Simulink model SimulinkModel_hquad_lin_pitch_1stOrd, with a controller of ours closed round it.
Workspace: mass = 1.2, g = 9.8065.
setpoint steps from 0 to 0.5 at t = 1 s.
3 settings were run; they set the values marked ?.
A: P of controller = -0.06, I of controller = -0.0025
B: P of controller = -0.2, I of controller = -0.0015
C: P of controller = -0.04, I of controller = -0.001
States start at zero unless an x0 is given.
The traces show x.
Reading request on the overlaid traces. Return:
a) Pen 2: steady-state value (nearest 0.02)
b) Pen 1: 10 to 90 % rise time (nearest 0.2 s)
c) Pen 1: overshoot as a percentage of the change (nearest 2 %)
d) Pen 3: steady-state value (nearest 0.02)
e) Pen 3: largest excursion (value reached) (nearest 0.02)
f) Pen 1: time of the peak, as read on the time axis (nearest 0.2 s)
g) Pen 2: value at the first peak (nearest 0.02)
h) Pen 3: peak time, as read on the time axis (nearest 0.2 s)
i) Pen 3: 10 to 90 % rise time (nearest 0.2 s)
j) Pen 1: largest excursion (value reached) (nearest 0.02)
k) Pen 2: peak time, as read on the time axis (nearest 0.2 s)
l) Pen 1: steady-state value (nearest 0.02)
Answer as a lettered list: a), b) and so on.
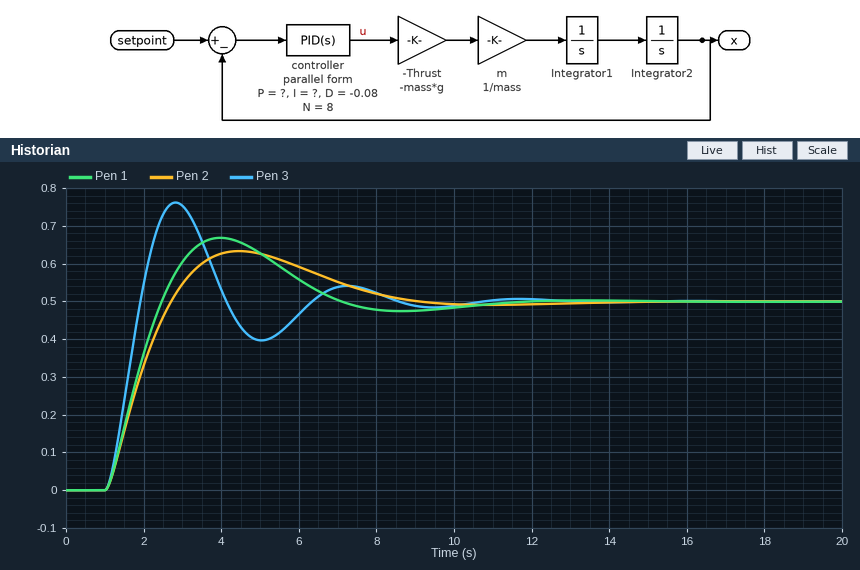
a) 0.50
b) 1.0 s
c) 34 %
d) 0.50
e) 0.76
f) 4.0 s
g) 0.64
h) 2.8 s
i) 0.6 s
j) 0.66
k) 4.4 s
l) 0.50
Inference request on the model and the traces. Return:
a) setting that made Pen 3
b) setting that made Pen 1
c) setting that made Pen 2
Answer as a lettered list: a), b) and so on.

a) B
b) A
c) C
